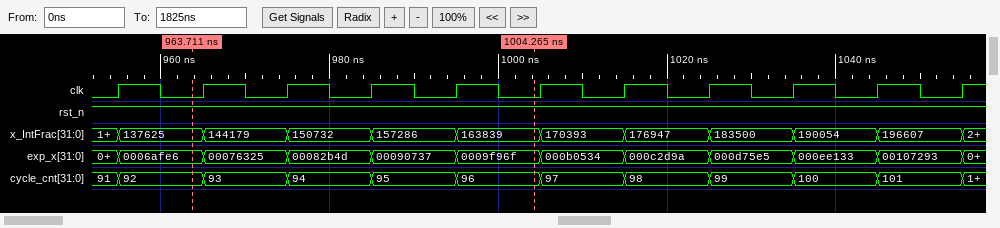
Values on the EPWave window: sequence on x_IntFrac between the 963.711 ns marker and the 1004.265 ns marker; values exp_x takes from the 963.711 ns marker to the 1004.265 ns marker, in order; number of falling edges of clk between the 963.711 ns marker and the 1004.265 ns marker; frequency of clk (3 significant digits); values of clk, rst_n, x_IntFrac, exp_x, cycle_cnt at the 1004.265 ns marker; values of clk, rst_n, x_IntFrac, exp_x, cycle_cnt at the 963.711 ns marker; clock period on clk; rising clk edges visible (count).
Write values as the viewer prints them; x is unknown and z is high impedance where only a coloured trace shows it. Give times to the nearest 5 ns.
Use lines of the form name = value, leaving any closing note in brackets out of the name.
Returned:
sequence on x_IntFrac between the 963.711 ns marker and the 1004.265 ns marker = 137625, 144179, 150732, 157286, 163839
values exp_x takes from the 963.711 ns marker to the 1004.265 ns marker, in order = 0006afe6, 00076325, 00082b4d, 00090737, 0009f96f
number of falling edges of clk between the 963.711 ns marker and the 1004.265 ns marker = 4
frequency of clk = 100 MHz
values of clk, rst_n, x_IntFrac, exp_x, cycle_cnt at the 1004.265 ns marker = clk=0, rst_n=1, x_IntFrac=163839, exp_x=0009f96f, cycle_cnt=96
values of clk, rst_n, x_IntFrac, exp_x, cycle_cnt at the 963.711 ns marker = clk=0, rst_n=1, x_IntFrac=137625, exp_x=0006afe6, cycle_cnt=92
clock period on clk = 10 ns
rising clk edges visible = 11
